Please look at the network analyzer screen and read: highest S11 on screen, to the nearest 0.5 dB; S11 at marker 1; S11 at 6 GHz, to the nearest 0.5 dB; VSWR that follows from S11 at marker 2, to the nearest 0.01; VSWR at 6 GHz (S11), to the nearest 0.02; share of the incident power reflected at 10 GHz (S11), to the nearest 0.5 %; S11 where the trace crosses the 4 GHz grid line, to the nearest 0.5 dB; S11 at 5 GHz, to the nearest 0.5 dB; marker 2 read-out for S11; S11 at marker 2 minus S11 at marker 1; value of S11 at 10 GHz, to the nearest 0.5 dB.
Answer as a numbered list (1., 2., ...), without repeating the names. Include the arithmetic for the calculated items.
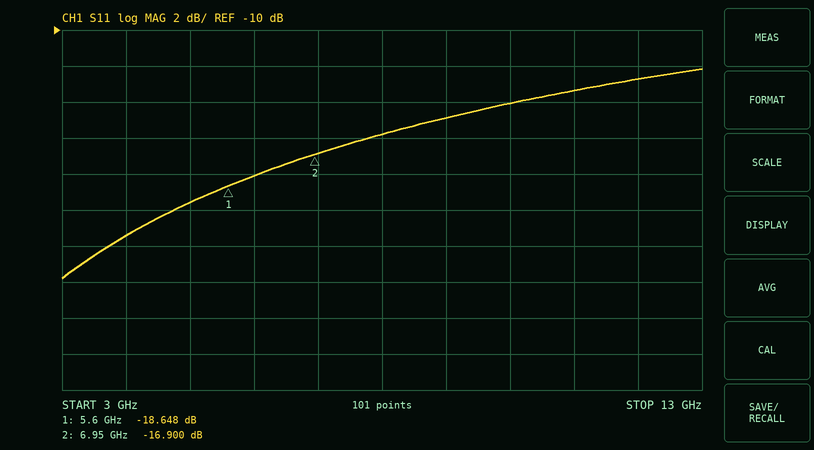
1. -12.0 dB
2. -18.648 dB
3. -18.0 dB
4. (1 + 0.1429)/(1 − 0.1429) ≈ 1.33
5. |Γ| = 10^(-18/20) = 0.1259; VSWR = (1 + 0.1259)/(1 − 0.1259) ≈ 1.29, so 1.28 to the nearest 0.02
6. 10^(-14/10) ≈ 4.0 %
7. -21.5 dB
8. -19.5 dB
9. -16.900 dB
10. -16.9 − (-18.648) = 1.748 dB
11. -14.0 dB
